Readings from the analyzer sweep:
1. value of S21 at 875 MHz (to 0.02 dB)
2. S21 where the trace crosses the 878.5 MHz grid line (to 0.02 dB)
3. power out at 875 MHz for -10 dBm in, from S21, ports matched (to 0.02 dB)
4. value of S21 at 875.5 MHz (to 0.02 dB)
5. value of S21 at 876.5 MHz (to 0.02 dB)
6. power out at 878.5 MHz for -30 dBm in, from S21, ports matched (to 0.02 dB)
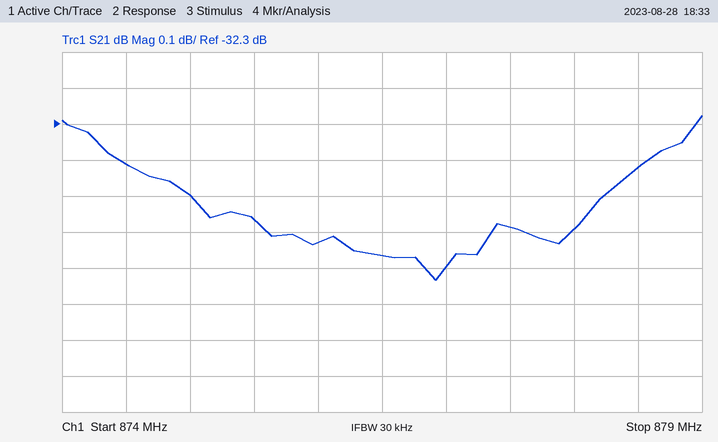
-32.50 dB
-32.42 dB
-42.50 dBm
-32.56 dB
-32.66 dB
-62.42 dBm
